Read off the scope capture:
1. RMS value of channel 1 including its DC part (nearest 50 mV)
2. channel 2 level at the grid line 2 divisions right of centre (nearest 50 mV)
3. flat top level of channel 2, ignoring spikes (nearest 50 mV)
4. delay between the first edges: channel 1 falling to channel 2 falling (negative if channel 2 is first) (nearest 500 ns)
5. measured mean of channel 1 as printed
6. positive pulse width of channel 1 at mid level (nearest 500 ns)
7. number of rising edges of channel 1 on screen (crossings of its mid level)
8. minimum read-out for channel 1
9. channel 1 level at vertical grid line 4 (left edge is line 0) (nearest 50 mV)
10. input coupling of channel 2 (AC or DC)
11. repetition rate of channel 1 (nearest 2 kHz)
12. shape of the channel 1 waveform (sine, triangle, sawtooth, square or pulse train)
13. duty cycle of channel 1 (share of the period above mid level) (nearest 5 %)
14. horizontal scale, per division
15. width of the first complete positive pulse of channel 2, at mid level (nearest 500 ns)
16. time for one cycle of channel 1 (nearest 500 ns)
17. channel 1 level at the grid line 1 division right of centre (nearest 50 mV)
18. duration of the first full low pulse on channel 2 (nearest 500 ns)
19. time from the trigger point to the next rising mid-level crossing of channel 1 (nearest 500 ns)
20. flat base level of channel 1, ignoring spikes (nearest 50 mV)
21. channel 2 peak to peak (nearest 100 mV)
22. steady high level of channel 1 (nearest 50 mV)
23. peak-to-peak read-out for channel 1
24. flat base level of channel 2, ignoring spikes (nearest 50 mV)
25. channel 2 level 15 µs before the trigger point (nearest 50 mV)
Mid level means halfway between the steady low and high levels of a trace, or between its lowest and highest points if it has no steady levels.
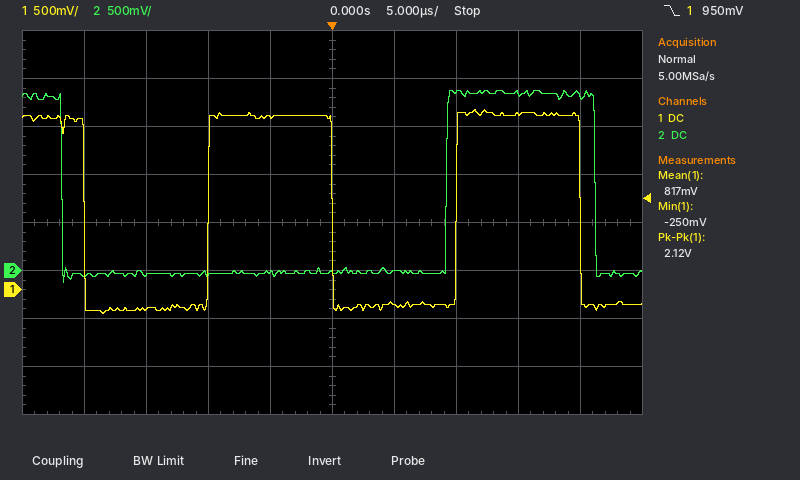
1.30 V
1.85 V
1.85 V
-2.0 µs
817 mV
10.0 µs
2
-250 mV
1.80 V
DC
50 kHz
square
50 %
5 µs
12.0 µs
20.0 µs
-150 mV
31.0 µs
10.0 µs
-200 mV
2.00 V
1.80 V
2.12 V
-50 mV
-50 mV
